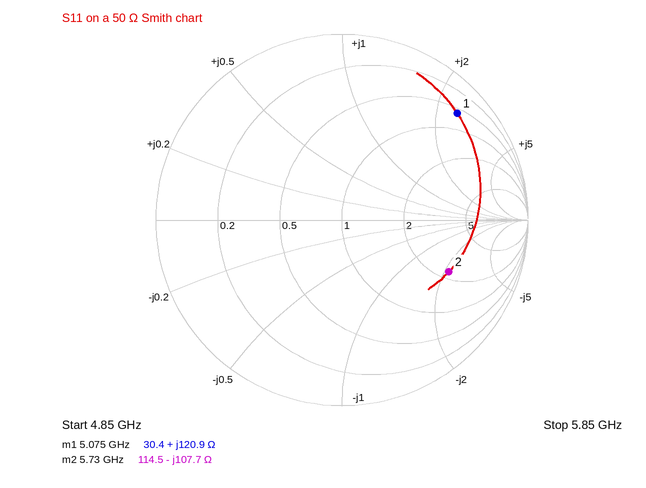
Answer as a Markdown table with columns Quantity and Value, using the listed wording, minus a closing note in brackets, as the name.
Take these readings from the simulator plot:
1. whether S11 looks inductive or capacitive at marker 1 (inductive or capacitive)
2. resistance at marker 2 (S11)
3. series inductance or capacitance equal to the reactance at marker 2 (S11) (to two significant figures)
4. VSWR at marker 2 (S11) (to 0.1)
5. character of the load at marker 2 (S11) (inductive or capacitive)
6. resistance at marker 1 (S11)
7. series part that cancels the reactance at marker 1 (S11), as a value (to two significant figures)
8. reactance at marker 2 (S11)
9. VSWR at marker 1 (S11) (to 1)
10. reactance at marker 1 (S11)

| Quantity | Value |
|---|---|
| whether S11 looks inductive or capacitive at marker 1 | inductive |
| resistance at marker 2 | 114.5 Ω |
| series inductance or capacitance equal to the reactance at marker 2 (S11) | 260 fF |
| VSWR at marker 2 (S11) | 4.5 |
| character of the load at marker 2 (S11) | capacitive |
| resistance at marker 1 | 30.4 Ω |
| series part that cancels the reactance at marker 1 (S11), as a value | 260 fF |
| reactance at marker 2 | -107.7 Ω |
| VSWR at marker 1 (S11) | 12 |
| reactance at marker 1 | +120.9 Ω |
